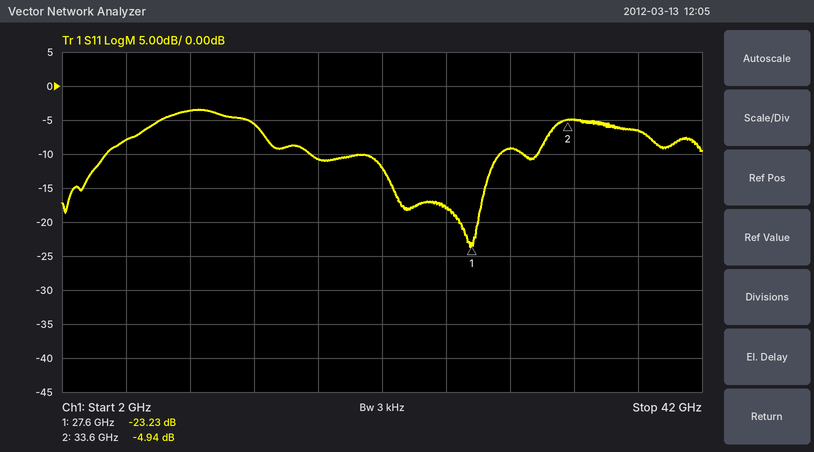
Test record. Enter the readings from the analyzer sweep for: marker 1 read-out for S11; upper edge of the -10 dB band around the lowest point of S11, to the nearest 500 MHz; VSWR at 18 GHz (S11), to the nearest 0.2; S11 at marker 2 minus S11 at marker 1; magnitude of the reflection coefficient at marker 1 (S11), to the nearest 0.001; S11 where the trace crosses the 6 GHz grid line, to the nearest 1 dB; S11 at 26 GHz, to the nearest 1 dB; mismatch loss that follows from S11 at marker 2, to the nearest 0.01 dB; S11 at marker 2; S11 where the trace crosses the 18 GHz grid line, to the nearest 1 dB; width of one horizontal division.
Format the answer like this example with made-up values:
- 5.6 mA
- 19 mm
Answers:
- -23.23 dB
- 29.5 GHz
- 1.8
- 18.29 dB
- 0.069
- -8 dB
- -18 dB
- 1.68 dB
- -4.94 dB
- -11 dB
- 4 GHz
